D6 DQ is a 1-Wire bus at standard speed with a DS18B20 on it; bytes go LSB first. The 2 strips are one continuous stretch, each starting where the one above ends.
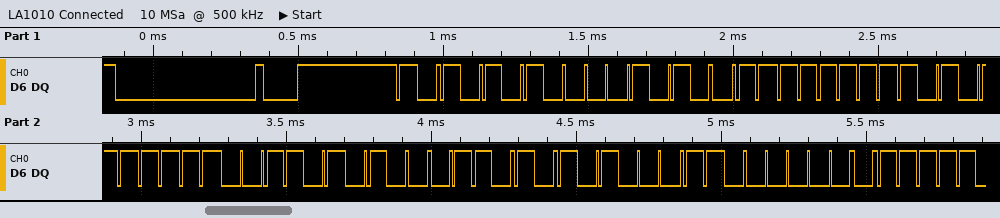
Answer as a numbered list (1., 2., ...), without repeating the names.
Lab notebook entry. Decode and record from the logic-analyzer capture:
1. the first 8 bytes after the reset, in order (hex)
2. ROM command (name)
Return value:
1. 55 28 FF F5 B3 62 15 03
2. Match ROM
